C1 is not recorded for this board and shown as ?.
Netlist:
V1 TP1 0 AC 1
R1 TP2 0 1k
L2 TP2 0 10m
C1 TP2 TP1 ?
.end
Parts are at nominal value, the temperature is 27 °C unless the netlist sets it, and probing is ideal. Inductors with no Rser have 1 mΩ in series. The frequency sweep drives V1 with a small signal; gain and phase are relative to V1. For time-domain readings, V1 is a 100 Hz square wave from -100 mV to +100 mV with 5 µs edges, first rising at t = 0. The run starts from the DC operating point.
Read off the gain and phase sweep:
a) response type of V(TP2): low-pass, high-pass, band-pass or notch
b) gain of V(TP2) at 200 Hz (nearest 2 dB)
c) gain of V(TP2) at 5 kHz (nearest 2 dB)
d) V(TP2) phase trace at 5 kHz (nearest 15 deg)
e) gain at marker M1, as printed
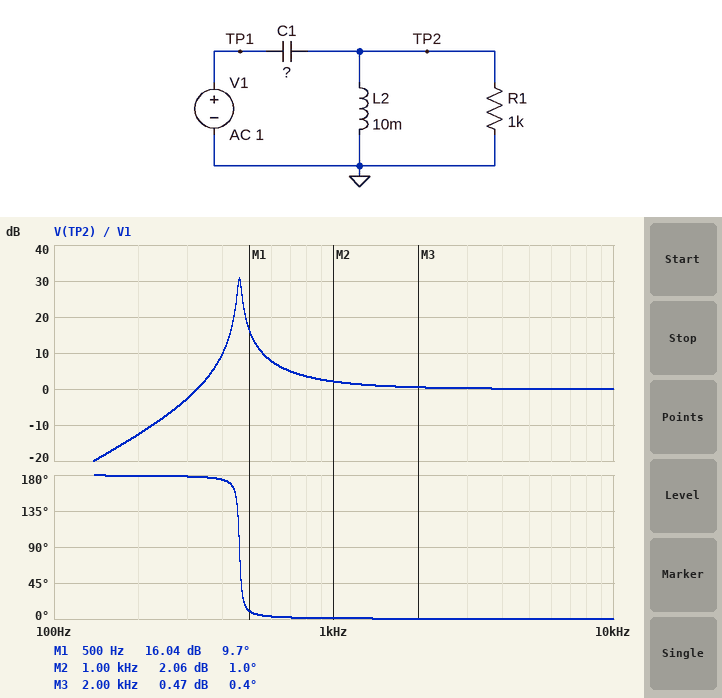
high-pass
-12 dB
0 dB
0 deg
16.04 dB
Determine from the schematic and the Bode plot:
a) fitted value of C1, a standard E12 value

12 µF
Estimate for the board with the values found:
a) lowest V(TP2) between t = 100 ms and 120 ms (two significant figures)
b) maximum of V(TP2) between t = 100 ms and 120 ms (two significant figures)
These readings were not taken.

-180 mV
180 mV
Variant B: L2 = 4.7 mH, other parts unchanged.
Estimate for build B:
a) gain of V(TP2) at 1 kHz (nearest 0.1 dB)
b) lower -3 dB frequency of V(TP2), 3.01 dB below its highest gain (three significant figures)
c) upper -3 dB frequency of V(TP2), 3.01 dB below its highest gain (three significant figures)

5.2 dB
664 Hz
677 Hz
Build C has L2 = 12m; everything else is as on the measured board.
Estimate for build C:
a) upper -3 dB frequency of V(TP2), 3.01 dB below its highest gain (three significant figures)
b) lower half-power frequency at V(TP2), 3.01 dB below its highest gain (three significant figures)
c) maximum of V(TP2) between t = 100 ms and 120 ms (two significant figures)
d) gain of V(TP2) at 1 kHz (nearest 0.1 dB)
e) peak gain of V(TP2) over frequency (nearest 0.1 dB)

426 Hz
413 Hz
120 mV
1.7 dB
30.0 dB
